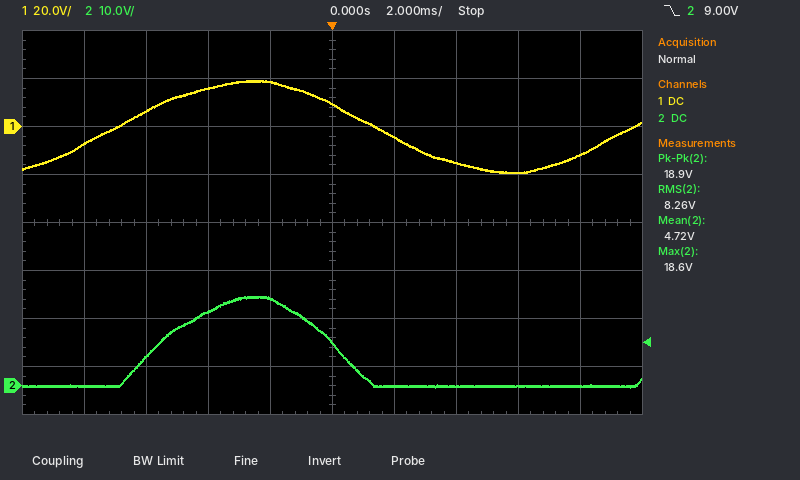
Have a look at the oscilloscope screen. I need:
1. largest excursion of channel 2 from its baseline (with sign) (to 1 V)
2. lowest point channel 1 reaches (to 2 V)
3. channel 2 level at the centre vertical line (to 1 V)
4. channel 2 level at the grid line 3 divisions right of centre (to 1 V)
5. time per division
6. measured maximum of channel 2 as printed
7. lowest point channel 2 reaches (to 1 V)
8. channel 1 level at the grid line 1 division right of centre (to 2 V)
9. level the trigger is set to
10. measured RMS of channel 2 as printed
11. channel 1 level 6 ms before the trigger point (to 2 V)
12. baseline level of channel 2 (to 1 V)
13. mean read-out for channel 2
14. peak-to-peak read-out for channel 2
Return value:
+19 V
-20 V
9 V
0 V
2 ms
18.6 V
0 V
-4 V
9.00 V
8.26 V
6 V
0 V
4.72 V
18.9 V
